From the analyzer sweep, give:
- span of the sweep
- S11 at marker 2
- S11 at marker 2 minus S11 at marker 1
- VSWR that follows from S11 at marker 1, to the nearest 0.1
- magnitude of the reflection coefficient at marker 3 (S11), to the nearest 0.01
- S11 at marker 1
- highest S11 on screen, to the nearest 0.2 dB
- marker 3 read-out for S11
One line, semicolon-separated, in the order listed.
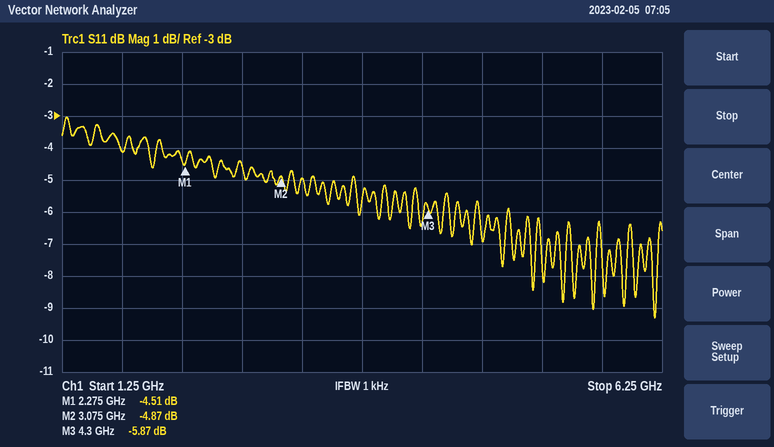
5 GHz; -4.87 dB; -0.36 dB; 3.9; 0.51; -4.51 dB; -3.0 dB; -5.87 dB
